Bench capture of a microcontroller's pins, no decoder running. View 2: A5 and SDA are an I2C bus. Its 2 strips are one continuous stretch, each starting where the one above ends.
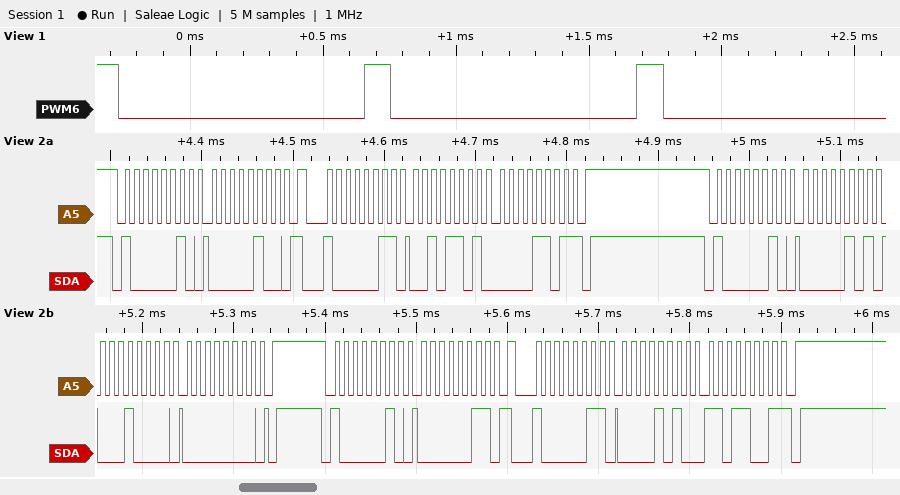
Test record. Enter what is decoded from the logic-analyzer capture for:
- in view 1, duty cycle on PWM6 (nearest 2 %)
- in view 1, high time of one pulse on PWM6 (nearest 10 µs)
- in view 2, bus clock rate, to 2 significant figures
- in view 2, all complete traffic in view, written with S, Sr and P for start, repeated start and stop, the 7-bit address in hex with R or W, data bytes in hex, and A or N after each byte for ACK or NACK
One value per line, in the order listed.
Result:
10 %
100 µs
100 kHz
S 41W A 04 A Sr 41R A 2D A 0D N P S 41W A 05 A 10 A 00 A P S 41W A 03 A Sr 41R A 0A A D9 N P
